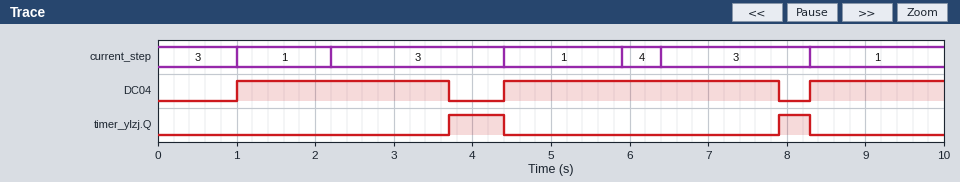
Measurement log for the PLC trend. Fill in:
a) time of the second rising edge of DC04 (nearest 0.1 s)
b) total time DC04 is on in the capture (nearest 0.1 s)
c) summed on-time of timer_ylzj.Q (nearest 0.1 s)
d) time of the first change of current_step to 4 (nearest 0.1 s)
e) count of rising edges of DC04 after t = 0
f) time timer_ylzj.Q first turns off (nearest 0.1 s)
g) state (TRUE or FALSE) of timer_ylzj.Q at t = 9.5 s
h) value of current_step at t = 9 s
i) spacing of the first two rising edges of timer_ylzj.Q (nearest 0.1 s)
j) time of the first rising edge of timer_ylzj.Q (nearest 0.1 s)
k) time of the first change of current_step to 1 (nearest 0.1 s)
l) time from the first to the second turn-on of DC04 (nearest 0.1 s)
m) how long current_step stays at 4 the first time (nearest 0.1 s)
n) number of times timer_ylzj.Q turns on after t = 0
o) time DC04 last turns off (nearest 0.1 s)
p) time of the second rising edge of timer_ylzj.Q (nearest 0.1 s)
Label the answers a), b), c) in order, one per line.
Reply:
a) 4.4 s
b) 7.9 s
c) 1.1 s
d) 5.9 s
e) 3
f) 4.4 s
g) FALSE
h) 1
i) 4.2 s
j) 3.7 s
k) 1.0 s
l) 3.4 s
m) 0.5 s
n) 2
o) 7.9 s
p) 7.9 s
